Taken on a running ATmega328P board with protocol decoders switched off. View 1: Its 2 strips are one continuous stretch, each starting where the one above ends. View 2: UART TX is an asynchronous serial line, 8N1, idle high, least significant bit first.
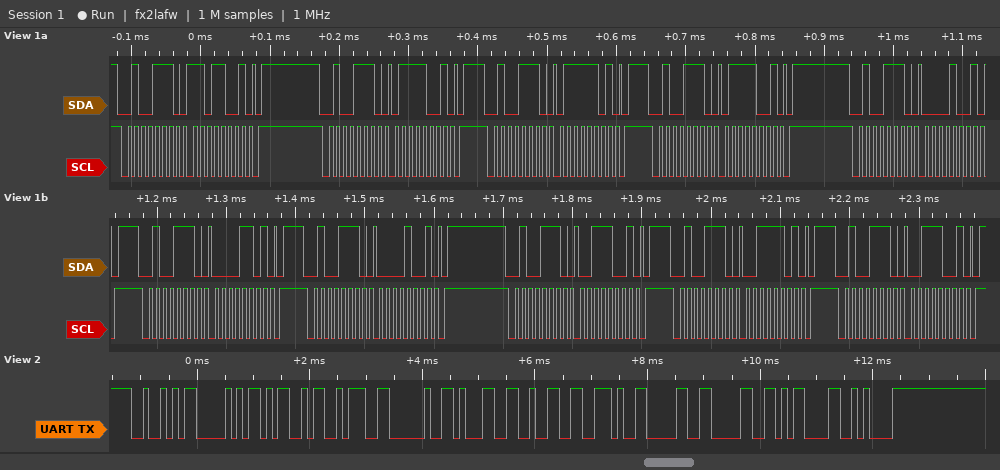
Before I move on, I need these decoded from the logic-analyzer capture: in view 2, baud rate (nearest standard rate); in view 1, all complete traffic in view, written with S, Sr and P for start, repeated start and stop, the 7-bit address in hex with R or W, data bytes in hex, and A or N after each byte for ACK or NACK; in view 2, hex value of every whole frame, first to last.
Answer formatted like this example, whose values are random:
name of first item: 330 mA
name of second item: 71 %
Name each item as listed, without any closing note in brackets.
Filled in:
in view 2, baud rate: 9600 baud
in view 1, all complete traffic in view, written with S, Sr and P for start, repeated start and stop, the 7-bit address in hex with R or W, data bytes in hex, and A or N after each byte for ACK or NACK: S 27W A D9 A P S 27W A 79 A P S 27W A 7D A P S 27W A 79 A P S 27W A 09 A P S 27W A 0D A P S 27W A 09 A P S 27W A 39 A P S 27W A 3D A P S 27W A 39 A P
in view 2, hex value of every whole frame, first to last: 52 50 4D 3A 20 31 32 2E 30 30 0D 0A
